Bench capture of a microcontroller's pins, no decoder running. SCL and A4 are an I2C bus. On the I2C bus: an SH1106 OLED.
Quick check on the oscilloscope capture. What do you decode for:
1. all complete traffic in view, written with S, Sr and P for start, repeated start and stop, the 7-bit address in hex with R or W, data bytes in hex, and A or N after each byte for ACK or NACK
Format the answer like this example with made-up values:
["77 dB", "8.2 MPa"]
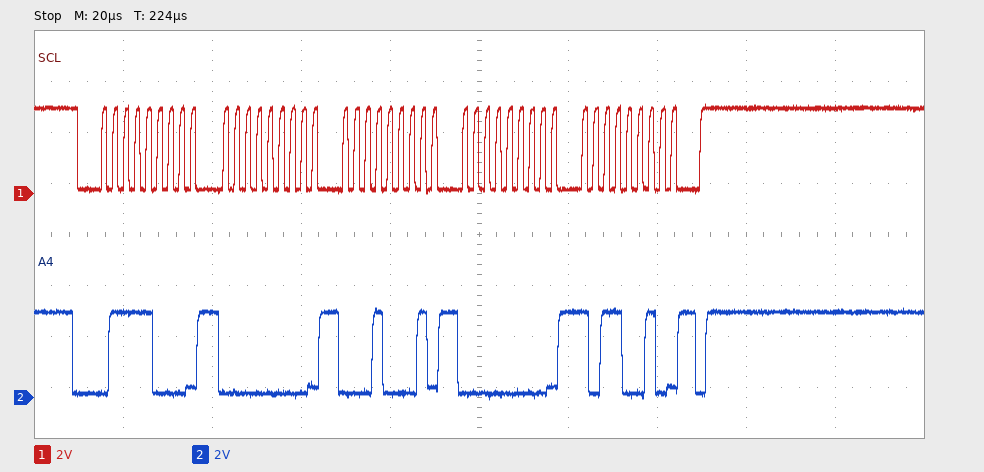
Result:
["S 3CW A 00 A 11 A 00 A B2 A P"]
